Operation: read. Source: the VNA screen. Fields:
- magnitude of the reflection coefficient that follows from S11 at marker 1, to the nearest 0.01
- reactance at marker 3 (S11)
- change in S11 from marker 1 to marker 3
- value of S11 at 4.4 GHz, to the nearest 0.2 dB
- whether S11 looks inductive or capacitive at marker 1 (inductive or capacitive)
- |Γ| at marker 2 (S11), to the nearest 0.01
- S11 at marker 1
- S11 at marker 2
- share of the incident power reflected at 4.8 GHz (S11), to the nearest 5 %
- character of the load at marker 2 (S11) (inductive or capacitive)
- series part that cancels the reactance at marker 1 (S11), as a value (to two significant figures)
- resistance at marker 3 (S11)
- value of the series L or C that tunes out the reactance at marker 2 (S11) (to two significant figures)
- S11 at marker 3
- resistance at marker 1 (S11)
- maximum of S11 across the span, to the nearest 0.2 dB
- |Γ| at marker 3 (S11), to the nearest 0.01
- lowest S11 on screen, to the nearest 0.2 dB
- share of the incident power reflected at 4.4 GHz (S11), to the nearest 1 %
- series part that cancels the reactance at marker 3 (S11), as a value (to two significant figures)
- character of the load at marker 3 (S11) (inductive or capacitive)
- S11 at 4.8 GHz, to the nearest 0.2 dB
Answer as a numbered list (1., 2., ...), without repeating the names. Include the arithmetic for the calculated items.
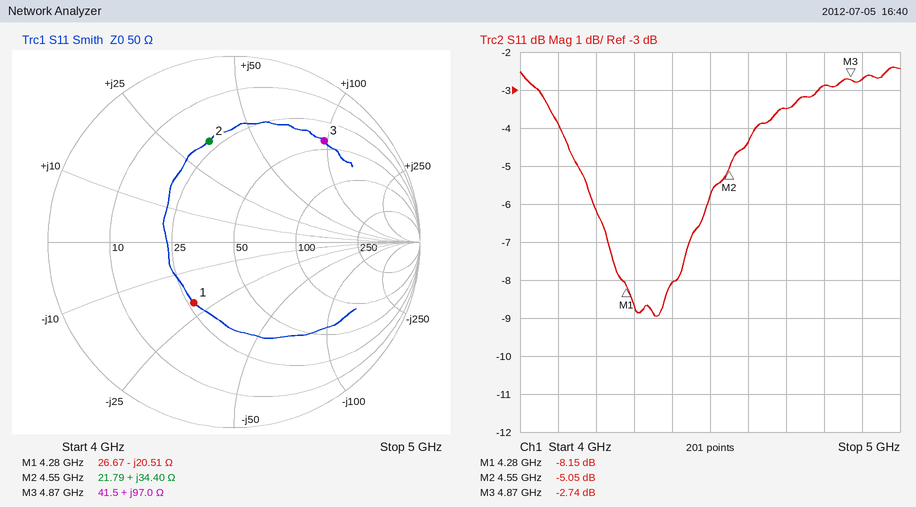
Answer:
1. 10^(-8.15/20) ≈ 0.39
2. +97.0 Ω
3. -2.74 − (-8.15) = 5.41 dB
4. -8.0 dB
5. capacitive
6. 0.56
7. -8.15 dB
8. -5.05 dB
9. 10^(-2.8/10) ≈ 52.5 %, so 50 % to the nearest 5 %
10. inductive
11. L = 20.51 Ω/(2π × 4.28 GHz) ≈ 763 pH, so 760 pH to two significant figures
12. 41.5 Ω
13. C = 1/(2π × 4.55 GHz × 34.4 Ω) ≈ 1.0 pF
14. -2.74 dB
15. 26.67 Ω
16. -2.4 dB
17. 0.73
18. -9.0 dB
19. 10^(-8/10) ≈ 16 %
20. C = 1/(2π × 4.87 GHz × 97 Ω) ≈ 337 fF, so 340 fF to two significant figures
21. inductive
22. -2.8 dB
